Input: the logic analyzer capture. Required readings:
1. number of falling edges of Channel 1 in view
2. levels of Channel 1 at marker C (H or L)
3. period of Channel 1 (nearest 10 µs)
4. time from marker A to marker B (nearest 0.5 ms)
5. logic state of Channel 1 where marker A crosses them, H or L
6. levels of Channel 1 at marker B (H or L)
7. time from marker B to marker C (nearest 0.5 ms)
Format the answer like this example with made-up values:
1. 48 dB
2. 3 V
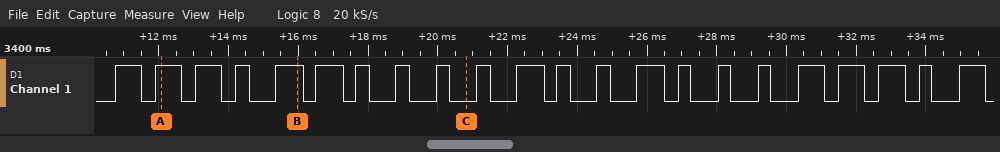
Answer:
1. 22
2. Channel 1=L
3. 1150 µs
4. 4 ms
5. Channel 1=H
6. Channel 1=H
7. 5 ms
